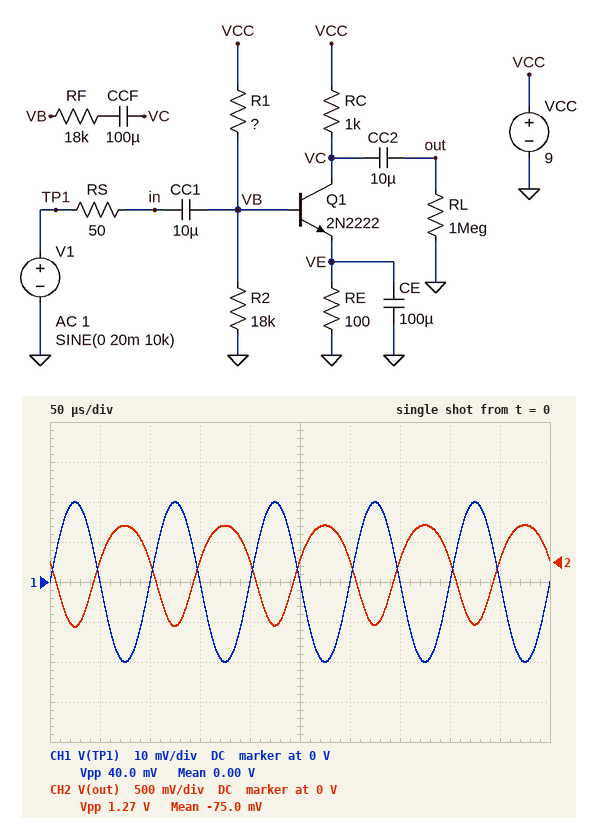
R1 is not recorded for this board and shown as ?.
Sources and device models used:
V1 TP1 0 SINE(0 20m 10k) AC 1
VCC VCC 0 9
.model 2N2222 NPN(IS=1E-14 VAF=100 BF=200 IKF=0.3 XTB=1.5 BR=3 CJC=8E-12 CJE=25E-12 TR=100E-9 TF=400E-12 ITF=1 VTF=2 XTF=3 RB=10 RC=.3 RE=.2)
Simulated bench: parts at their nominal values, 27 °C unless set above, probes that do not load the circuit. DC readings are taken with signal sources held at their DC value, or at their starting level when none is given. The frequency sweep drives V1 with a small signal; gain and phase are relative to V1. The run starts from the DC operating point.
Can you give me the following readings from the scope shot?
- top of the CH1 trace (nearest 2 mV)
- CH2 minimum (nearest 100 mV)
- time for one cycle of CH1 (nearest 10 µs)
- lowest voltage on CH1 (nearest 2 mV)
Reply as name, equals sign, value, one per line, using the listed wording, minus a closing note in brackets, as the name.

top of the CH1 trace = 20 mV
CH2 minimum = -800 mV
time for one cycle of CH1 = 100 µs
lowest voltage on CH1 = -20 mV
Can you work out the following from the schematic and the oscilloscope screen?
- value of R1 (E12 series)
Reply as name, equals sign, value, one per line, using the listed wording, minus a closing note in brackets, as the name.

value of R1 = 180 kΩ
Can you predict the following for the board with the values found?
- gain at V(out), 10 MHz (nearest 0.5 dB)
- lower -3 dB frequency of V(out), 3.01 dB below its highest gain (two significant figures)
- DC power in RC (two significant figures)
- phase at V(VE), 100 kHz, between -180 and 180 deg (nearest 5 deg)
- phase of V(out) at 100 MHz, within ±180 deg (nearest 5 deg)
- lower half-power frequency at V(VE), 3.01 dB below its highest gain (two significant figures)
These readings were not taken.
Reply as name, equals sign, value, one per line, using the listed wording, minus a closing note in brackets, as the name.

gain at V(out), 10 MHz = 27.5 dB
lower -3 dB frequency of V(out), 3.01 dB below its highest gain = 90 Hz
DC power in RC = 880 µW
phase at V(VE), 100 kHz, between -180 and 180 deg = -90 deg
phase of V(out) at 100 MHz, within ±180 deg = 65 deg
lower half-power frequency at V(VE), 3.01 dB below its highest gain = 5.7 Hz
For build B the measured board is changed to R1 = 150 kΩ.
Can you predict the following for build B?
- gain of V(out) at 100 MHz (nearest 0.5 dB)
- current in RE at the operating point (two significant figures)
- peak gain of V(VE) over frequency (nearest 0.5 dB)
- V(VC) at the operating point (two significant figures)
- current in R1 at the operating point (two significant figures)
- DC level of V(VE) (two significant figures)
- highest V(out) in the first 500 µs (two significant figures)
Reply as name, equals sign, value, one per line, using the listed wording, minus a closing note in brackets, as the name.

gain of V(out) at 100 MHz = 12.5 dB
current in RE at the operating point = 1.7 mA
peak gain of V(VE) over frequency = -5.0 dB
V(VC) at the operating point = 7.3 V
current in R1 at the operating point = 54 µA
DC level of V(VE) = 170 mV
highest V(out) in the first 500 µs = 800 mV
